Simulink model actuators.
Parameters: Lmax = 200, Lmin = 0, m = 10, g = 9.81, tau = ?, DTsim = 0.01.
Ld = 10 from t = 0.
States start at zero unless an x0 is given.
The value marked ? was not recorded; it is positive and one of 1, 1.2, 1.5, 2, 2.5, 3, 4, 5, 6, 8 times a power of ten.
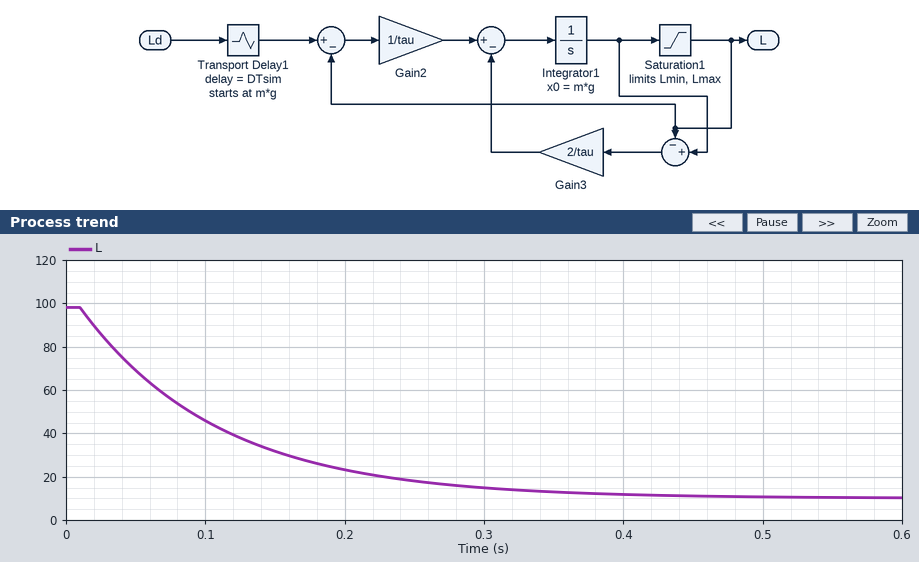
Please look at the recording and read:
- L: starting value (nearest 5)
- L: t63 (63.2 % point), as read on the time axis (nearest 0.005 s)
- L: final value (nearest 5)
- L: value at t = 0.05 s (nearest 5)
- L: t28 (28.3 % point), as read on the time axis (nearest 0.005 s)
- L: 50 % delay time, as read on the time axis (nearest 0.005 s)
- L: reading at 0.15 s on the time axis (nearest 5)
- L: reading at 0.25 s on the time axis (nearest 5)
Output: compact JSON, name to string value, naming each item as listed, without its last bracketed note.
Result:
{"L: starting value": "100", "L: t63 (63.2 % point), as read on the time axis": "0.110 s", "L: final value": "10", "L: value at t = 0.05 s": "70", "L: t28 (28.3 % point), as read on the time axis": "0.045 s", "L: 50 % delay time, as read on the time axis": "0.080 s", "L: reading at 0.15 s on the time axis": "30", "L: reading at 0.25 s on the time axis": "20"}
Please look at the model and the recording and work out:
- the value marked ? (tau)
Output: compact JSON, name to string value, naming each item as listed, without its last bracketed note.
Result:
{"the value marked ?": "0.1"}
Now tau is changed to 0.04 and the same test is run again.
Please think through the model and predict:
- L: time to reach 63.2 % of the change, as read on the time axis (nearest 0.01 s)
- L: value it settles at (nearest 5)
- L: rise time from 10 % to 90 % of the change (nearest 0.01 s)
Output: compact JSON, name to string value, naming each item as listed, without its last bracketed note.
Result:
{"L: time to reach 63.2 % of the change, as read on the time axis": "0.05 s", "L: value it settles at": "10", "L: rise time from 10 % to 90 % of the change": "0.09 s"}
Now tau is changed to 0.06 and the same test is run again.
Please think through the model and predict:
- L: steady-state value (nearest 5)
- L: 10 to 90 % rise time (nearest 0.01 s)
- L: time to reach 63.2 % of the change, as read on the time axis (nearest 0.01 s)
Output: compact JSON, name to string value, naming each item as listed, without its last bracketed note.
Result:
{"L: steady-state value": "10", "L: 10 to 90 % rise time": "0.13 s", "L: time to reach 63.2 % of the change, as read on the time axis": "0.07 s"}
